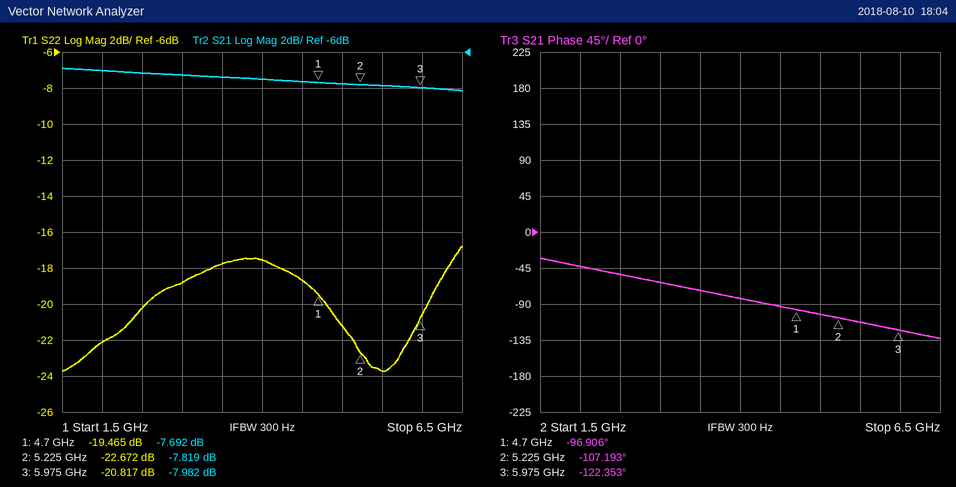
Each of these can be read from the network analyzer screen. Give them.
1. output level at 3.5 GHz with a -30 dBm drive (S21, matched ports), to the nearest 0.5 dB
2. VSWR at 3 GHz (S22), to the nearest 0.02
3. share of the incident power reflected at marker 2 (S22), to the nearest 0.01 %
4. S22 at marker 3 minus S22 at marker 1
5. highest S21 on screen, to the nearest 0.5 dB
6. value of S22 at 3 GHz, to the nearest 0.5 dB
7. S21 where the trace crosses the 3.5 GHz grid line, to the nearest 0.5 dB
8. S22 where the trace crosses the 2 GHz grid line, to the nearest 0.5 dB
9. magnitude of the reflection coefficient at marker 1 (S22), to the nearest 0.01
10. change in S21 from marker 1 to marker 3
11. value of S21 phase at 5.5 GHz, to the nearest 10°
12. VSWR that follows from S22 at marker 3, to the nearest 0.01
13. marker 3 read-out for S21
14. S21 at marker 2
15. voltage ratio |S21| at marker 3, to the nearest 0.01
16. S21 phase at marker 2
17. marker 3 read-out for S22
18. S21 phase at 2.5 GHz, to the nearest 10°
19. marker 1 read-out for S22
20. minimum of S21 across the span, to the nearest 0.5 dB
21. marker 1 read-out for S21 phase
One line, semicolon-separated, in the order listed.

-37.5 dBm; 1.26; 0.54 %; -1.352 dB; -7.0 dB; -19.0 dB; -7.5 dB; -22.0 dB; 0.11; -0.290 dB; -110°; 1.20; -7.982 dB; -7.819 dB; 0.40; -107.193°; -20.817 dB; -50°; -19.465 dB; -8.0 dB; -96.906°
